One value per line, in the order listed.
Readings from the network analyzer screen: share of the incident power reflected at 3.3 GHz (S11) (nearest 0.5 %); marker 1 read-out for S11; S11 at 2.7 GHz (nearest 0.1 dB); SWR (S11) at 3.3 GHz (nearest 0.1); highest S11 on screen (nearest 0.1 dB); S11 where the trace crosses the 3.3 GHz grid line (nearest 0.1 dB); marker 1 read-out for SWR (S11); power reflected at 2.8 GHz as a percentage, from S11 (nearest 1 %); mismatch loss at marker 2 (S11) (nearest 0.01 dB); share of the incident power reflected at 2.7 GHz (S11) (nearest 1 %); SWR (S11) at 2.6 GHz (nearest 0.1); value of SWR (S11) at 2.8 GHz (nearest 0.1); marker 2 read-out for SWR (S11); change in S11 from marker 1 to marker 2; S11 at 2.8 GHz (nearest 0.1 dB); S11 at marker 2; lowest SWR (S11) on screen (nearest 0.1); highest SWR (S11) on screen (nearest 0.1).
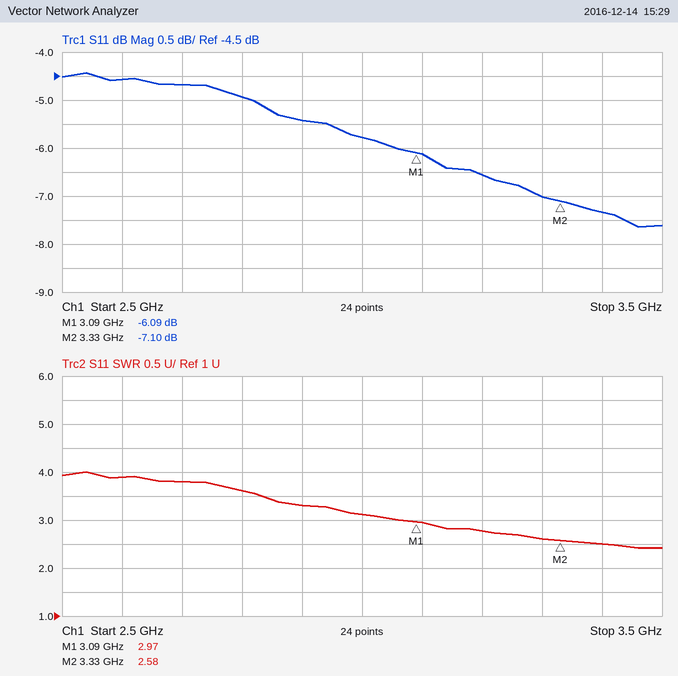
20.0 %
-6.09 dB
-4.7 dB
2.6
-4.4 dB
-7.0 dB
2.97
32 %
0.94 dB
34 %
3.9
3.6
2.58
-1.01 dB
-4.9 dB
-7.10 dB
2.4
4.0
